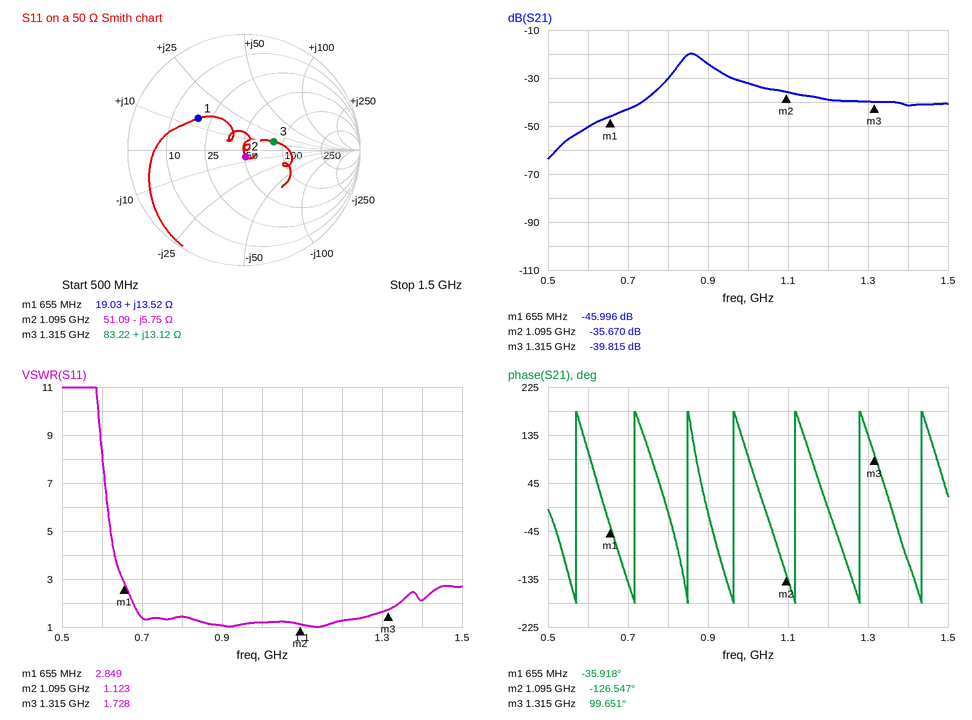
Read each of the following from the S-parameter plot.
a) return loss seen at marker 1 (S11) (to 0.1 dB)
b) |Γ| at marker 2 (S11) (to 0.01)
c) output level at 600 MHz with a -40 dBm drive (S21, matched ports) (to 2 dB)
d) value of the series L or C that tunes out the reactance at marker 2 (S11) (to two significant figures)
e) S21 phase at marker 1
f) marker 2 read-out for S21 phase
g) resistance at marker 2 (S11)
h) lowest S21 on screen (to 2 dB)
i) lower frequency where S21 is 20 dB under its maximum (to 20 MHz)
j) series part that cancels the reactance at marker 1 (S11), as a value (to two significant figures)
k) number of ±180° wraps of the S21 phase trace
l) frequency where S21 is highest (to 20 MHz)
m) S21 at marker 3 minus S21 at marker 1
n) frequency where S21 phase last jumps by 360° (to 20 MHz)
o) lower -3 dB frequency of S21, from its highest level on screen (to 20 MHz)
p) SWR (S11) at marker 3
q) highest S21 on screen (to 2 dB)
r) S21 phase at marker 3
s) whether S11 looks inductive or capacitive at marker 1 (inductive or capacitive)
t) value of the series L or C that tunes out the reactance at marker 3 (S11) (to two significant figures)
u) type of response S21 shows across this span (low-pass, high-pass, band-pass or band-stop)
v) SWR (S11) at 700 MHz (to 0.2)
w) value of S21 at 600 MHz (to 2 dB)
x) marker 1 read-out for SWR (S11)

6.4 dB
0.06
-90 dBm
840 pH
-35.918°
-126.547°
51.09 Ω
-64 dB
740 MHz
18 pF
7
860 MHz
6.181 dB
1.44 GHz
840 MHz
1.728
-20 dB
99.651°
inductive
9.2 pF
band-pass
1.4
-50 dB
2.849
